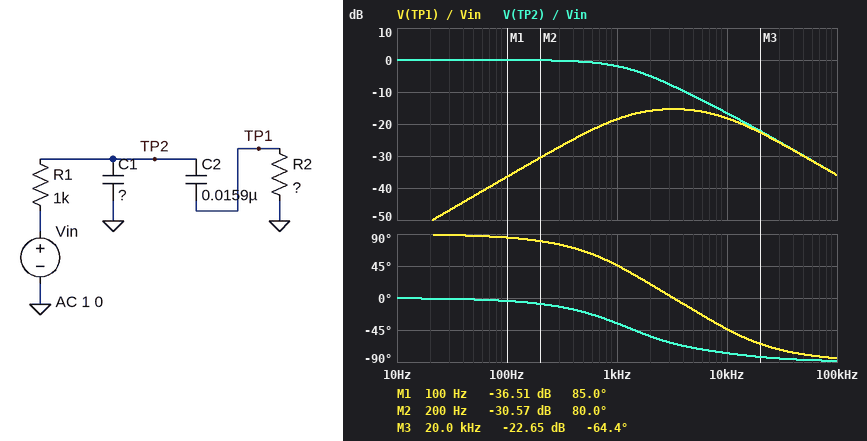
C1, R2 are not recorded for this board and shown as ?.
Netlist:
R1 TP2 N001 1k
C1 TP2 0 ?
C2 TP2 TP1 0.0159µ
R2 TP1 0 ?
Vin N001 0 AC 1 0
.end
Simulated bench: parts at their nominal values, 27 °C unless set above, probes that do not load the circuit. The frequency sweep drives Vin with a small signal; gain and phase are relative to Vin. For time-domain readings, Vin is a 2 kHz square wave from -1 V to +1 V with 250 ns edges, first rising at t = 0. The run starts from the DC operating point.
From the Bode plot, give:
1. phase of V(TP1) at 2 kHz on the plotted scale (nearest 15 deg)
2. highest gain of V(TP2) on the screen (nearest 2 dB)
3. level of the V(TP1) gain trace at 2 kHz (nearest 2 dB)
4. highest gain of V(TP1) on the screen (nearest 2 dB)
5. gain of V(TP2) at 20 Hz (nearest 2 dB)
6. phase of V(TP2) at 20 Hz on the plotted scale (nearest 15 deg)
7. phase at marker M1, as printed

15 deg
0 dB
-16 dB
-16 dB
0 dB
0 deg
85.0 deg
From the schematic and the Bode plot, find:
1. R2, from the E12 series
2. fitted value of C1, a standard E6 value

1.5 kΩ
100 nF
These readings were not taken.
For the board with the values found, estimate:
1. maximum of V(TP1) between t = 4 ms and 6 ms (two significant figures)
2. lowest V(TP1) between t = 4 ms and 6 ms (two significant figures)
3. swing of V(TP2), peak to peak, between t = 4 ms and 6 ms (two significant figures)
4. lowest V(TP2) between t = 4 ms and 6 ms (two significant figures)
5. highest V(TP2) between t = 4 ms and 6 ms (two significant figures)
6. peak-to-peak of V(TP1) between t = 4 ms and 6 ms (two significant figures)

240 mV
-240 mV
1.6 V
-790 mV
790 mV
480 mV
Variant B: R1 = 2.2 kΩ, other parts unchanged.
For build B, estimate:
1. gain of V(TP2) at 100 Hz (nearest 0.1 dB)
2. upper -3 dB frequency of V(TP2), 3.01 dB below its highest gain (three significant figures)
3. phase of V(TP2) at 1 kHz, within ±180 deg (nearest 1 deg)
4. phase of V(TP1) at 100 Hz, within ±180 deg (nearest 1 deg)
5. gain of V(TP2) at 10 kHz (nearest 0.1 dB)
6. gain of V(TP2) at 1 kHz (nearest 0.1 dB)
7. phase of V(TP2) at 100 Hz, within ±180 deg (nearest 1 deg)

-0.1 dB
617 Hz
-57 deg
80 deg
-23.3 dB
-5.6 dB
-9 deg
